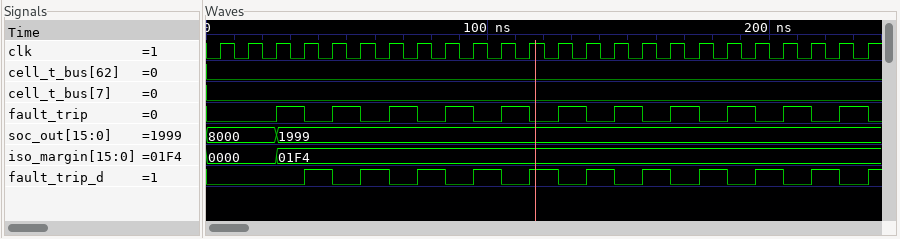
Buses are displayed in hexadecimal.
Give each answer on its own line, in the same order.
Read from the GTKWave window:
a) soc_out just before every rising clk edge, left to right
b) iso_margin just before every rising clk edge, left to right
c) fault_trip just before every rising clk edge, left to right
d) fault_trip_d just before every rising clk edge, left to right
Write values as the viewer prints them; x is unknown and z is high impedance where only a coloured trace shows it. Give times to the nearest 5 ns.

8000, 8000, 8000, 1999, 1999, 1999, 1999, 1999, 1999, 1999, 1999, 1999, 1999, 1999, 1999, 1999, 1999, 1999, 1999, 1999, 1999, 1999, 1999, 1999
0000, 0000, 0000, 01F4, 01F4, 01F4, 01F4, 01F4, 01F4, 01F4, 01F4, 01F4, 01F4, 01F4, 01F4, 01F4, 01F4, 01F4, 01F4, 01F4, 01F4, 01F4, 01F4, 01F4
0 0 0 1 0 1 0 1 0 1 0 1 0 1 0 1 0 1 0 1 0 1 0 1
0 0 0 0 1 0 1 0 1 0 1 0 1 0 1 0 1 0 1 0 1 0 1 0
